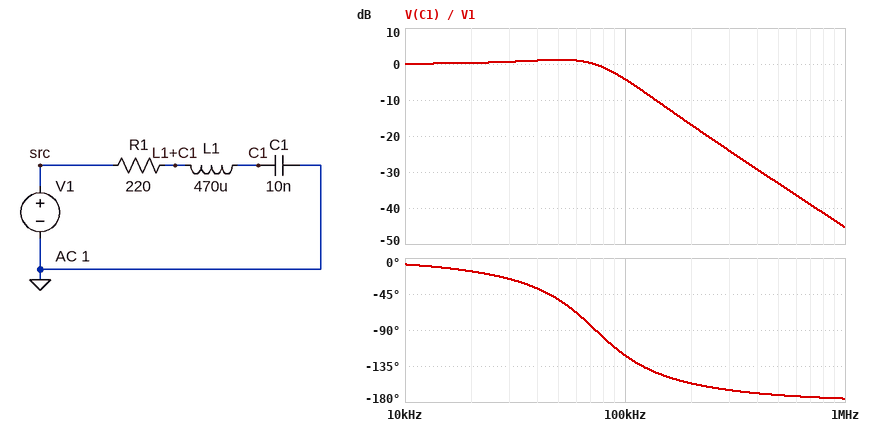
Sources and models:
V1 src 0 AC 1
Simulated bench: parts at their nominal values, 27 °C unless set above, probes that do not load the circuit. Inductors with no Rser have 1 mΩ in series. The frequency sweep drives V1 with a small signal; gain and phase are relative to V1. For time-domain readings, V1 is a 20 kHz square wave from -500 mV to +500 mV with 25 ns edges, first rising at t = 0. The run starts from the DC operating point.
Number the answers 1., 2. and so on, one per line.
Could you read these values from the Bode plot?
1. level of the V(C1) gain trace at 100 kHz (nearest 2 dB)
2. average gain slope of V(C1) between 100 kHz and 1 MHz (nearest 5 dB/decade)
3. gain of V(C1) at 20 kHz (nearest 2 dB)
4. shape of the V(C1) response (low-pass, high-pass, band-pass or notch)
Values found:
1. -4 dB
2. -40 dB/decade
3. 0 dB
4. low-pass
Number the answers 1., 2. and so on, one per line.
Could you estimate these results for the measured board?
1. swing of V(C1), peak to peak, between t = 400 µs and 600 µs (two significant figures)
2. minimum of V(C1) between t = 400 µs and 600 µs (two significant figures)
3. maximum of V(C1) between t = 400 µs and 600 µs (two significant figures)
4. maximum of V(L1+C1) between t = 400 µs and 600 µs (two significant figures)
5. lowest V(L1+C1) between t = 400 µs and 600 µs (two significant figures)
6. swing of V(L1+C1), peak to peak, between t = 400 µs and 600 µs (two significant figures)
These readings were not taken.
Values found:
1. 1.3 V
2. -660 mV
3. 660 mV
4. 590 mV
5. -590 mV
6. 1.2 V
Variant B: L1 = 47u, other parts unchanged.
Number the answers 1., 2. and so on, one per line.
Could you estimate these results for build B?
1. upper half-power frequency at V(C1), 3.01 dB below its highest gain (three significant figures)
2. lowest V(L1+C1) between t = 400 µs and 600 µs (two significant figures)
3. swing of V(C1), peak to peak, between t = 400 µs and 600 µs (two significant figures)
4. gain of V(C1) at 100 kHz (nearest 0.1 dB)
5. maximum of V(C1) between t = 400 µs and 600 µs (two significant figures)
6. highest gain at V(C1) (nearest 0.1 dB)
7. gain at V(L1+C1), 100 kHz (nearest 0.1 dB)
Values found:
1. 80.0 kHz
2. -500 mV
3. 1.0 V
4. -4.1 dB
5. 500 mV
6. 0 dB
7. -5.9 dB
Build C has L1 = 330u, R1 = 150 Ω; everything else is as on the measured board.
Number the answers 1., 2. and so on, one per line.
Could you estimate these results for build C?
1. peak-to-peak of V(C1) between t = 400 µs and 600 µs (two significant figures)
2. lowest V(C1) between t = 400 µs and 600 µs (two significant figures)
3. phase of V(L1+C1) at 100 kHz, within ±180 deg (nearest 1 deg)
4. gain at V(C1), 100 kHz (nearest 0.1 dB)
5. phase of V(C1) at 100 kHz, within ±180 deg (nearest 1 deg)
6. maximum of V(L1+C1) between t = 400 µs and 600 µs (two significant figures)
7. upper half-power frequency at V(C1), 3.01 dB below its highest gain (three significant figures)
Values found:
1. 1.5 V
2. -740 mV
3. 72 deg
4. 0.1 dB
5. -108 deg
6. 620 mV
7. 104 kHz
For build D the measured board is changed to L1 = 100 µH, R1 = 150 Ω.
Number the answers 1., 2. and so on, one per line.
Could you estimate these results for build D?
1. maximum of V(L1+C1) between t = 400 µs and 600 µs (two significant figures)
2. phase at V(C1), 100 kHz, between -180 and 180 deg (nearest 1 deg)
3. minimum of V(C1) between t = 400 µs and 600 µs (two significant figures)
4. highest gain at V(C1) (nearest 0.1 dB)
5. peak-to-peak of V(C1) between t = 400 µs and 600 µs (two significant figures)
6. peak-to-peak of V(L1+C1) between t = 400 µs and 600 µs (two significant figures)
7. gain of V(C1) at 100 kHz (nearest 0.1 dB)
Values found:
1. 520 mV
2. -57 deg
3. -530 mV
4. 0 dB
5. 1.1 V
6. 1.0 V
7. -1.0 dB
